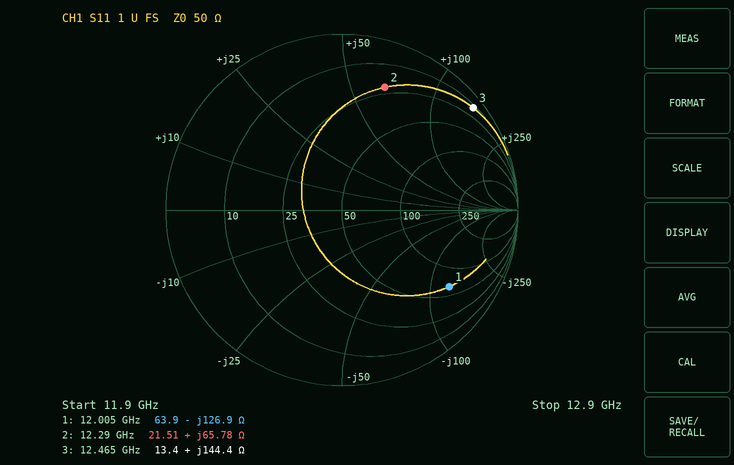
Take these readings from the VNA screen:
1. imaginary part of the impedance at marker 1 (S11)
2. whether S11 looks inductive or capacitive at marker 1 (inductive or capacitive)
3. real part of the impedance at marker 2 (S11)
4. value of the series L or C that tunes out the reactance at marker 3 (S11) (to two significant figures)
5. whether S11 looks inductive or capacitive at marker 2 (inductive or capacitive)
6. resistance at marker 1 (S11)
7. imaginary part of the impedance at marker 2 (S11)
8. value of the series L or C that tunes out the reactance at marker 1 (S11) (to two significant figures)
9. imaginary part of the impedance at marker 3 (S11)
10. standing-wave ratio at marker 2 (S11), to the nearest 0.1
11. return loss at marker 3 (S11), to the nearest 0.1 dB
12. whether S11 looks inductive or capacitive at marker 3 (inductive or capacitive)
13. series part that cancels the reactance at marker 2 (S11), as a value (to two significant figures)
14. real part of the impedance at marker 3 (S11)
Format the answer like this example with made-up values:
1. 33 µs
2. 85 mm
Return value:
1. -126.9 Ω
2. capacitive
3. 21.51 Ω
4. 88 fF
5. inductive
6. 63.9 Ω
7. +65.78 Ω
8. 1.7 nH
9. +144.4 Ω
10. 6.6
11. 0.5 dB
12. inductive
13. 200 fF
14. 13.4 Ω
